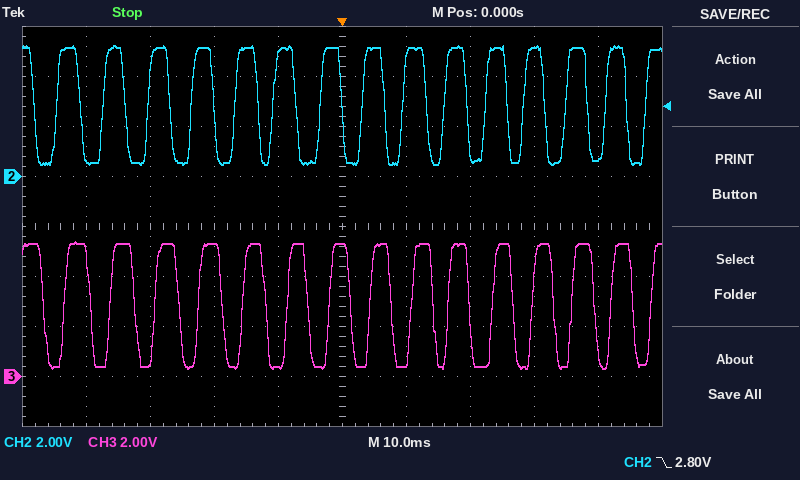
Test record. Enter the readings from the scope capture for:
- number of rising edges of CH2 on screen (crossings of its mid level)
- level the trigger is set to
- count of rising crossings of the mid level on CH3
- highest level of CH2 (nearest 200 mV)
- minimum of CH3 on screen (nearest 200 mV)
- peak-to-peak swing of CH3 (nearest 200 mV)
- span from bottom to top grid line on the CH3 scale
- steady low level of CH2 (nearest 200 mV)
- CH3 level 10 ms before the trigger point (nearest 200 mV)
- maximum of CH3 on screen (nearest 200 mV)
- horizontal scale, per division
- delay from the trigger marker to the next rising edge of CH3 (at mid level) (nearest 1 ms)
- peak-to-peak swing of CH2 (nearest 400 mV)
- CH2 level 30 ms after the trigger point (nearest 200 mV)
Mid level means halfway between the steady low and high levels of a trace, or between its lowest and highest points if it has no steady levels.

15
2.80 V
15
5.2 V
400 mV
5.0 V
16 V
600 mV
400 mV
5.4 V
10 ms
4 ms
4.8 V
5.2 V
